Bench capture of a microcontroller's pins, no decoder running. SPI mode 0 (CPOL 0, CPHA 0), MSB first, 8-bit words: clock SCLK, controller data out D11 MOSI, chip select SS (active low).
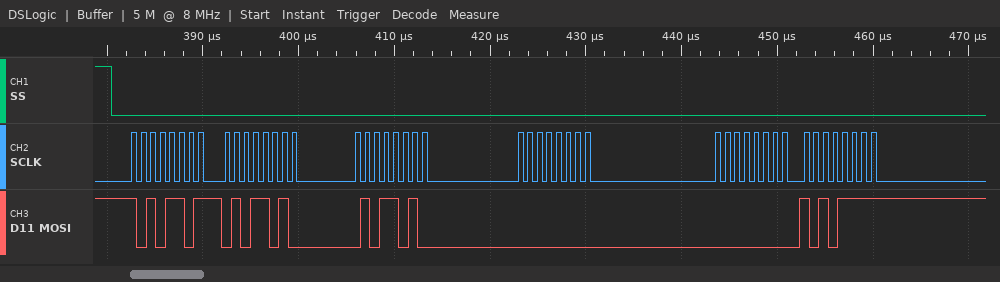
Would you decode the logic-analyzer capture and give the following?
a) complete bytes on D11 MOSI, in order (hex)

AD 5A 5A 00 00 AF
